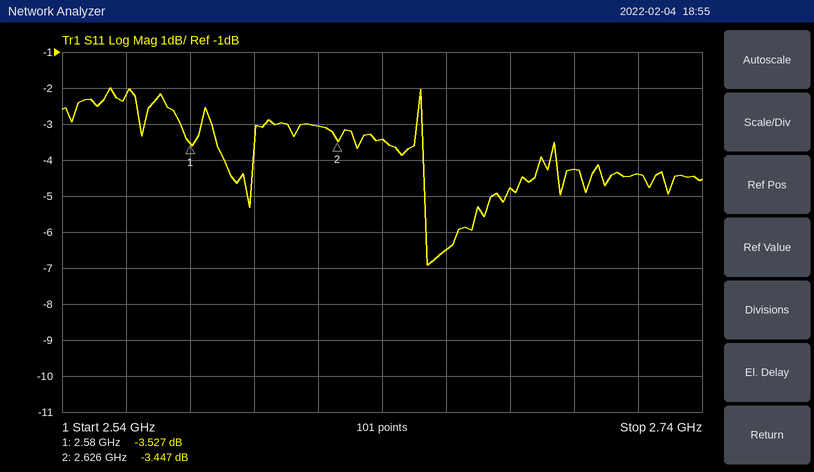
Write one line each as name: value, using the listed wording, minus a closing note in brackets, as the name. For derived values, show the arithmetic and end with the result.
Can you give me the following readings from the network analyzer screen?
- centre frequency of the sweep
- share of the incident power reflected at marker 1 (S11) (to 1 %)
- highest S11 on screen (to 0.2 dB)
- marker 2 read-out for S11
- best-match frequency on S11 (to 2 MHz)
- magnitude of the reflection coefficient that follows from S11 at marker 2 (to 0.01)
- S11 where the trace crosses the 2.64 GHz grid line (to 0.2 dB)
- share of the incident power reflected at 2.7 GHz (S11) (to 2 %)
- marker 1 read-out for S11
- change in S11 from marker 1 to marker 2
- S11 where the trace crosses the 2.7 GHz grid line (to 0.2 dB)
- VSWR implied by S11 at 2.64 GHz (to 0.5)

centre frequency of the sweep: 2.64 GHz
share of the incident power reflected at marker 1 (S11): 10^(-3.527/10) ≈ 44 %
highest S11 on screen: -2.0 dB
marker 2 read-out for S11: -3.447 dB
best-match frequency on S11: 2.654 GHz
magnitude of the reflection coefficient that follows from S11 at marker 2: 10^(-3.447/20) ≈ 0.67
S11 where the trace crosses the 2.64 GHz grid line: -3.4 dB
share of the incident power reflected at 2.7 GHz (S11): 10^(-4.2/10) ≈ 38 %
marker 1 read-out for S11: -3.527 dB
change in S11 from marker 1 to marker 2: -3.447 − (-3.527) = 0.080 dB
S11 where the trace crosses the 2.7 GHz grid line: -4.2 dB
VSWR implied by S11 at 2.64 GHz: |Γ| = 10^(-3.4/20) = 0.6761; VSWR = (1 + 0.6761)/(1 − 0.6761) ≈ 5.17, so 5.0 to the nearest 0.5
